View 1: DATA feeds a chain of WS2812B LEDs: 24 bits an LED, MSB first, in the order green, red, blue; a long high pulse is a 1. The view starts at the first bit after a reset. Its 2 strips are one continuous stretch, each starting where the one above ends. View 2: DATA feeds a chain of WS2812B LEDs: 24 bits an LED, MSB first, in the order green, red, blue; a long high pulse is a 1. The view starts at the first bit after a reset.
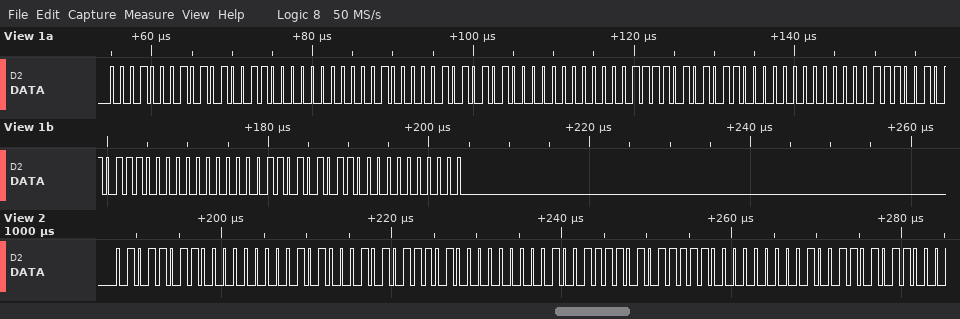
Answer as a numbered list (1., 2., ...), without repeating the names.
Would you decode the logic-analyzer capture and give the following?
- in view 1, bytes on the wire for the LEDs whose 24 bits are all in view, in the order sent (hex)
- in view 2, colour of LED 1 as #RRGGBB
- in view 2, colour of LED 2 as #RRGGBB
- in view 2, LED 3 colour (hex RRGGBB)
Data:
1. 11 53 00 10 55 00 0F 56 00 0E 57 00 0D 58 00
2. #005B51
3. #005D4F
4. #005F4D
